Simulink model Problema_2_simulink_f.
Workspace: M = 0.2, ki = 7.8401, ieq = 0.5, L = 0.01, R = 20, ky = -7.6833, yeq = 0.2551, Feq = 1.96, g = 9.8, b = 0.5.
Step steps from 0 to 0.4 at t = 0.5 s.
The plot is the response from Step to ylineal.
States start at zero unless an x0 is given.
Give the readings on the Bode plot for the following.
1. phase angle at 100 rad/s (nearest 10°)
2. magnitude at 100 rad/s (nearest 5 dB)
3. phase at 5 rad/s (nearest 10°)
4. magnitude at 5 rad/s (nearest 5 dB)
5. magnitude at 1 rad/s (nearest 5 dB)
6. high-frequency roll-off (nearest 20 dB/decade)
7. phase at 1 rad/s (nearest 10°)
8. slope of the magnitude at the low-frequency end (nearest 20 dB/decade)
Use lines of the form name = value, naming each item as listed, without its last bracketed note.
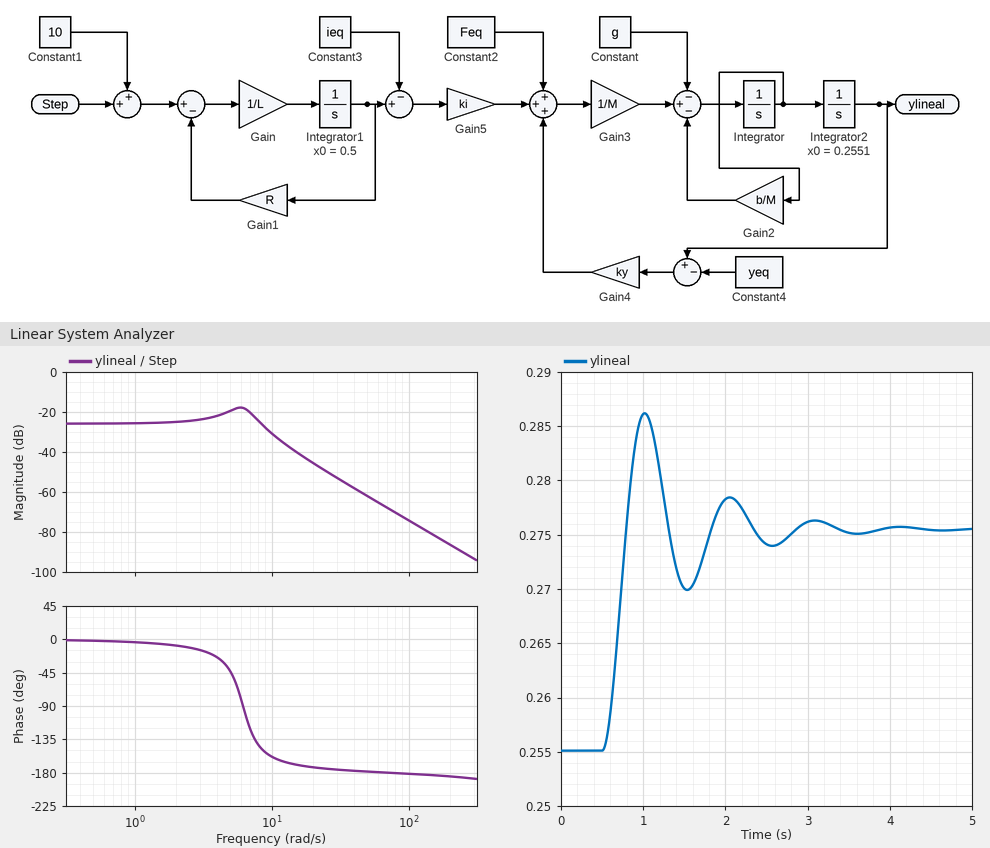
phase angle at 100 rad/s = -180°
magnitude at 100 rad/s = -75 dB
phase at 5 rad/s = -40°
magnitude at 5 rad/s = -20 dB
magnitude at 1 rad/s = -25 dB
high-frequency roll-off = -40 dB/decade
phase at 1 rad/s = 0°
slope of the magnitude at the low-frequency end = 0 dB/decade
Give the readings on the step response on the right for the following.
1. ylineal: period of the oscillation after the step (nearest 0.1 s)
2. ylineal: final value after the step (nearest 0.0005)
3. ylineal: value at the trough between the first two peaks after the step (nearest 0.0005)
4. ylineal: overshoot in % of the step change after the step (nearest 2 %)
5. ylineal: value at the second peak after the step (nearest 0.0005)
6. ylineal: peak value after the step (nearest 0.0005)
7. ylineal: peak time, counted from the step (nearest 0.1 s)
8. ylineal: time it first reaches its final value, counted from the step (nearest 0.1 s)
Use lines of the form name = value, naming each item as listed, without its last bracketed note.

ylineal: period of the oscillation after the step = 1.0 s
ylineal: final value after the step = 0.2755
ylineal: value at the trough between the first two peaks after the step = 0.2700
ylineal: overshoot in % of the step change after the step = 52 %
ylineal: value at the second peak after the step = 0.2785
ylineal: peak value after the step = 0.2860
ylineal: peak time, counted from the step = 0.5 s
ylineal: time it first reaches its final value, counted from the step = 0.3 s
